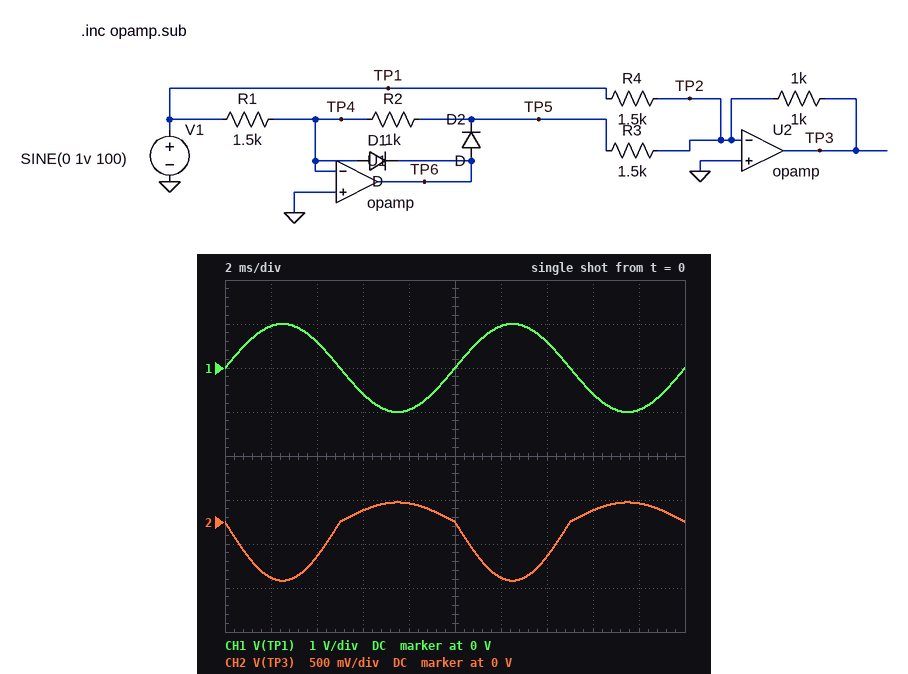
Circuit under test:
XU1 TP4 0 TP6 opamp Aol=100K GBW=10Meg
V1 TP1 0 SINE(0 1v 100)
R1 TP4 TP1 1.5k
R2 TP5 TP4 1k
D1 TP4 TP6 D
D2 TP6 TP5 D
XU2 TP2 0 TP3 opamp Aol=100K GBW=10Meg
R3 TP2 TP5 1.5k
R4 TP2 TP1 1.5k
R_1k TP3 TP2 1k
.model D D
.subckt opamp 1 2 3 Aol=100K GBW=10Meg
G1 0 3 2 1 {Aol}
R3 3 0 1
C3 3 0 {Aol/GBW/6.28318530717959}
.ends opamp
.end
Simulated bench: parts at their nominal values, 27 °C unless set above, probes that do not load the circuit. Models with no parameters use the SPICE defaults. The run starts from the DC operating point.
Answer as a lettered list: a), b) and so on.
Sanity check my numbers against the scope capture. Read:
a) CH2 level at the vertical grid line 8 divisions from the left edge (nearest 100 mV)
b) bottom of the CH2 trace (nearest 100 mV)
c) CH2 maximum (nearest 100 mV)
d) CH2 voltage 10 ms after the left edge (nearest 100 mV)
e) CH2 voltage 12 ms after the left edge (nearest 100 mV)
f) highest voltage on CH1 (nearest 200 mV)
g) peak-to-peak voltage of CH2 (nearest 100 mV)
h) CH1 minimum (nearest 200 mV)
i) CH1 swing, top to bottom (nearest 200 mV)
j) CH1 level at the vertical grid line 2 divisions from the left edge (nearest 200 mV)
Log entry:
a) 100 mV
b) -700 mV
c) 200 mV
d) 0 V
e) -600 mV
f) 1.0 V
g) 900 mV
h) -1.0 V
i) 2.0 V
j) 600 mV
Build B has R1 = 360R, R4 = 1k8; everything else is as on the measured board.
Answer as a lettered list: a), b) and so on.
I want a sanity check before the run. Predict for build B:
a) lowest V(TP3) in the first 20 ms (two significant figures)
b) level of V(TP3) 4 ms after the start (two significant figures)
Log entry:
a) -1.3 V
b) -330 mV
